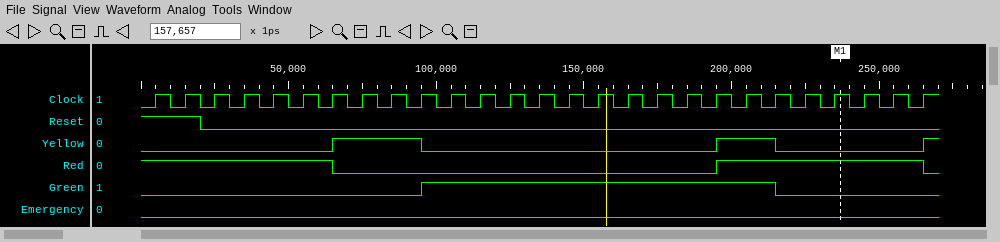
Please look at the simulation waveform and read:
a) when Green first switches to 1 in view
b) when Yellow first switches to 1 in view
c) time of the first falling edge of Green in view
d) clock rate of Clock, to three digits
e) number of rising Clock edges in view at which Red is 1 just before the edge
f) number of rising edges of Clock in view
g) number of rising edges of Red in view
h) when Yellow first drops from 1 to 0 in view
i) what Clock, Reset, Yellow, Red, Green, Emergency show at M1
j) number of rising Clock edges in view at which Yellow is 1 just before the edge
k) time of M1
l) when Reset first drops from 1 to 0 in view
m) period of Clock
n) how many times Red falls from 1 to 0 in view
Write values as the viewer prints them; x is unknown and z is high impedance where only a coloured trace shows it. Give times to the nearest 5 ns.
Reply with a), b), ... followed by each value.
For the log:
a) 95 ns
b) 65 ns
c) 215 ns
d) 100 MHz
e) 14
f) 27
g) 1
h) 95 ns
i) Clock=1, Reset=0, Yellow=0, Red=1, Green=0, Emergency=0
j) 5
k) 235 ns
l) 20 ns
m) 10 ns
n) 2
